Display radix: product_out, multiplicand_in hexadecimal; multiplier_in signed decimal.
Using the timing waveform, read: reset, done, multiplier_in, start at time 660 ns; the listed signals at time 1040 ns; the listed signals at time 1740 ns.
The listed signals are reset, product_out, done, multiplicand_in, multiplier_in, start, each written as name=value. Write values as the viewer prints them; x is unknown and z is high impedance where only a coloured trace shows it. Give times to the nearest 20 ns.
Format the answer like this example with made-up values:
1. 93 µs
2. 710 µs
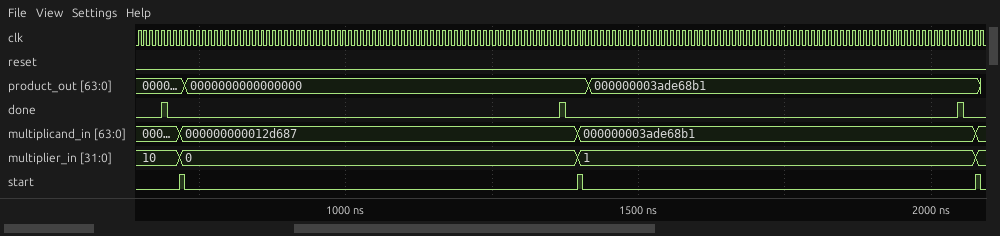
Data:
1. reset=0, done=0, multiplier_in=10, start=0
2. reset=0, product_out=0000000000000000, done=0, multiplicand_in=000000000012d687, multiplier_in=0, start=0
3. reset=0, product_out=000000003ade68b1, done=0, multiplicand_in=000000003ade68b1, multiplier_in=1, start=0
